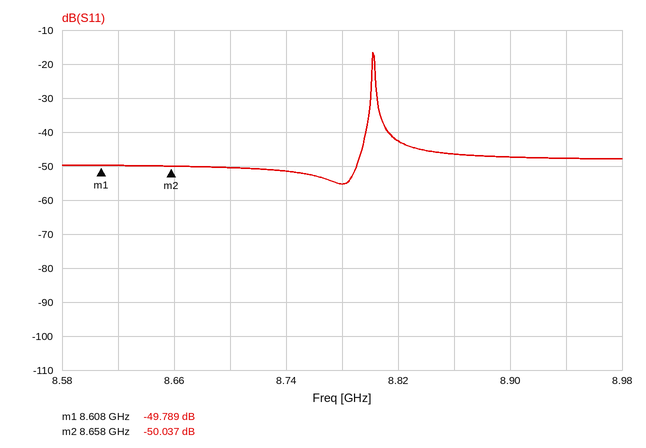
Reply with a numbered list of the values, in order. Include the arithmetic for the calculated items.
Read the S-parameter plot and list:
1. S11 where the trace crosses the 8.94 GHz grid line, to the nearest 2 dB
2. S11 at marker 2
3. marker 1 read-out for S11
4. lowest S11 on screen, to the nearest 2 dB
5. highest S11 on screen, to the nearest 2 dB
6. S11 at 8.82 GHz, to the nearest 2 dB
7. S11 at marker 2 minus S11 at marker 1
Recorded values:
1. -48 dB
2. -50.037 dB
3. -49.789 dB
4. -56 dB
5. -16 dB
6. -42 dB
7. -50.037 − (-49.789) = -0.248 dB
